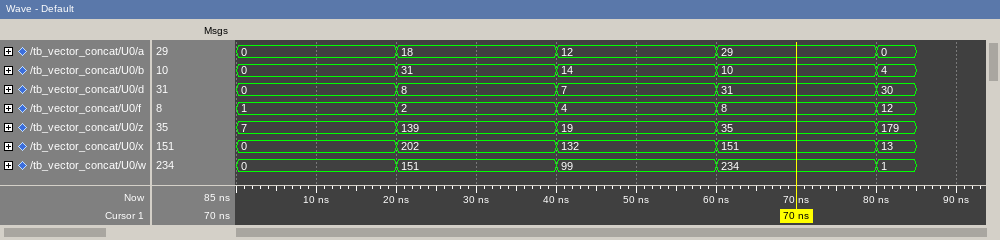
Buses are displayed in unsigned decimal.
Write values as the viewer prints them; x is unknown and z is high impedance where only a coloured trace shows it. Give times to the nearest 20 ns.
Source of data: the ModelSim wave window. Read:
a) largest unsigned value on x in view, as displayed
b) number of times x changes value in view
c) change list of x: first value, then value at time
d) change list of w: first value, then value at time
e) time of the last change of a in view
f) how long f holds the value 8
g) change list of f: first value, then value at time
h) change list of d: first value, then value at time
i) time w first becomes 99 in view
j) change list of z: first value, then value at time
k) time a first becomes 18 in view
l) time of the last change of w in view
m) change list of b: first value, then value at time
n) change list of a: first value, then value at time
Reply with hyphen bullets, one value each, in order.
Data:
- 202
- 4
- 0, 202 at 20 ns, 132 at 40 ns, 151 at 60 ns, 13 at 80 ns
- 0, 151 at 20 ns, 99 at 40 ns, 234 at 60 ns, 1 at 80 ns
- 80 ns
- 20 ns
- 1, 2 at 20 ns, 4 at 40 ns, 8 at 60 ns, 12 at 80 ns
- 0, 8 at 20 ns, 7 at 40 ns, 31 at 60 ns, 30 at 80 ns
- 40 ns
- 7, 139 at 20 ns, 19 at 40 ns, 35 at 60 ns, 179 at 80 ns
- 20 ns
- 80 ns
- 0, 31 at 20 ns, 14 at 40 ns, 10 at 60 ns, 4 at 80 ns
- 0, 18 at 20 ns, 12 at 40 ns, 29 at 60 ns, 0 at 80 ns
